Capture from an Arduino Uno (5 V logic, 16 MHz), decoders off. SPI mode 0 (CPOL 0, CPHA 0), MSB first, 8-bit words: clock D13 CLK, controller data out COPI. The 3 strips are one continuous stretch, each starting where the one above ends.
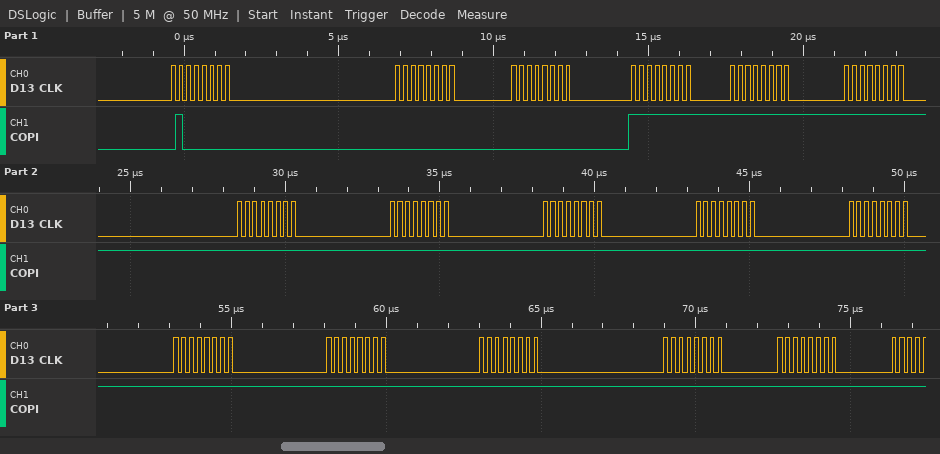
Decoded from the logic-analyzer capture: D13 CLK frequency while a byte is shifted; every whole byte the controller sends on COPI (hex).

4 MHz
40 00 00 FF FF FF FF FF FF FF FF FF FF FF FF FF
